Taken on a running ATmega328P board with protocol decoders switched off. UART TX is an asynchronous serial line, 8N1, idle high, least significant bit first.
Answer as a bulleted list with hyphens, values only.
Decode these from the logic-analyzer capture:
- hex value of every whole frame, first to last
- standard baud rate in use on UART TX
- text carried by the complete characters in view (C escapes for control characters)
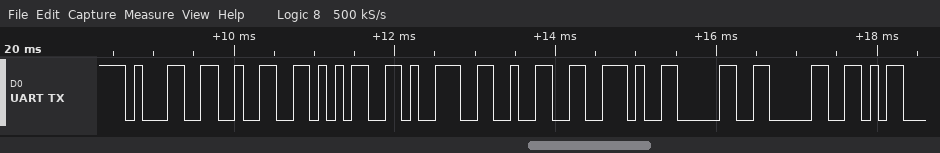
- 0x31 0x32 0x35 0x39 0x32 0x2E 0x30 0x30
- 9600 baud
- "12592.00"
